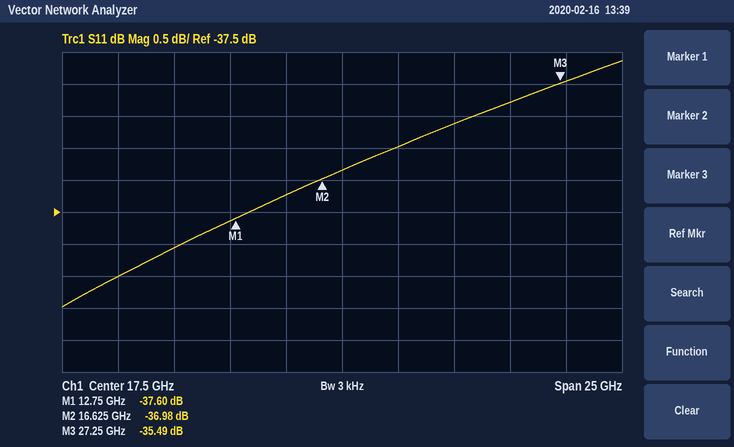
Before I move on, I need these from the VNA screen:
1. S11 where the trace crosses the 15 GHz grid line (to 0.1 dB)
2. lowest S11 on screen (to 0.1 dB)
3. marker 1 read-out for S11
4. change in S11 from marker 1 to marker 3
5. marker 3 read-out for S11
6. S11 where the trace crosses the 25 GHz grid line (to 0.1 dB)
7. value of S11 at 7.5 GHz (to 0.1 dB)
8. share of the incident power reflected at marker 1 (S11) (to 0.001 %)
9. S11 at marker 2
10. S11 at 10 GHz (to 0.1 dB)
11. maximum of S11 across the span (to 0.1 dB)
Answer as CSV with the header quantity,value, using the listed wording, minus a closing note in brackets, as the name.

quantity,value
S11 where the trace crosses the 15 GHz grid line,-37.2 dB
lowest S11 on screen,-39.0 dB
marker 1 read-out for S11,-37.60 dB
change in S11 from marker 1 to marker 3,2.11 dB
marker 3 read-out for S11,-35.49 dB
S11 where the trace crosses the 25 GHz grid line,-35.8 dB
value of S11 at 7.5 GHz,-38.5 dB
share of the incident power reflected at marker 1 (S11),0.017 %
S11 at marker 2,-36.98 dB
S11 at 10 GHz,-38.1 dB
maximum of S11 across the span,-35.1 dB
